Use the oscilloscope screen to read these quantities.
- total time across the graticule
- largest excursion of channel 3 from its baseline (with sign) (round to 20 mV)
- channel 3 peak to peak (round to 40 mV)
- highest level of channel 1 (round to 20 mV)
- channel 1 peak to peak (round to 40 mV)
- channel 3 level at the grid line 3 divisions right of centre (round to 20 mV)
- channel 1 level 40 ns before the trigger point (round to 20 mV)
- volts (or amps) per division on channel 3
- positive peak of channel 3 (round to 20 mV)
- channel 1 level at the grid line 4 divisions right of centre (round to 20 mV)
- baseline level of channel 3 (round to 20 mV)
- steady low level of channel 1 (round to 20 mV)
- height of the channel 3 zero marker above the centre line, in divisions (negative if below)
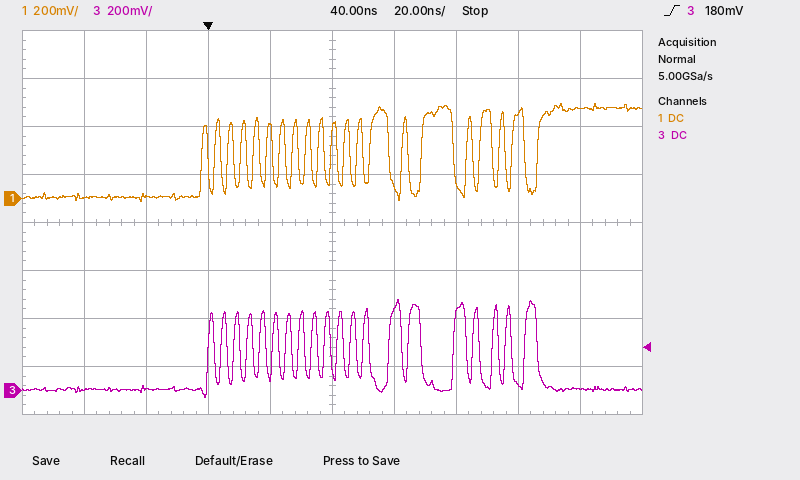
200 ns
+380 mV
400 mV
400 mV
400 mV
20 mV
0 mV
200 mV
380 mV
380 mV
0 mV
0 mV
-3.5 div
